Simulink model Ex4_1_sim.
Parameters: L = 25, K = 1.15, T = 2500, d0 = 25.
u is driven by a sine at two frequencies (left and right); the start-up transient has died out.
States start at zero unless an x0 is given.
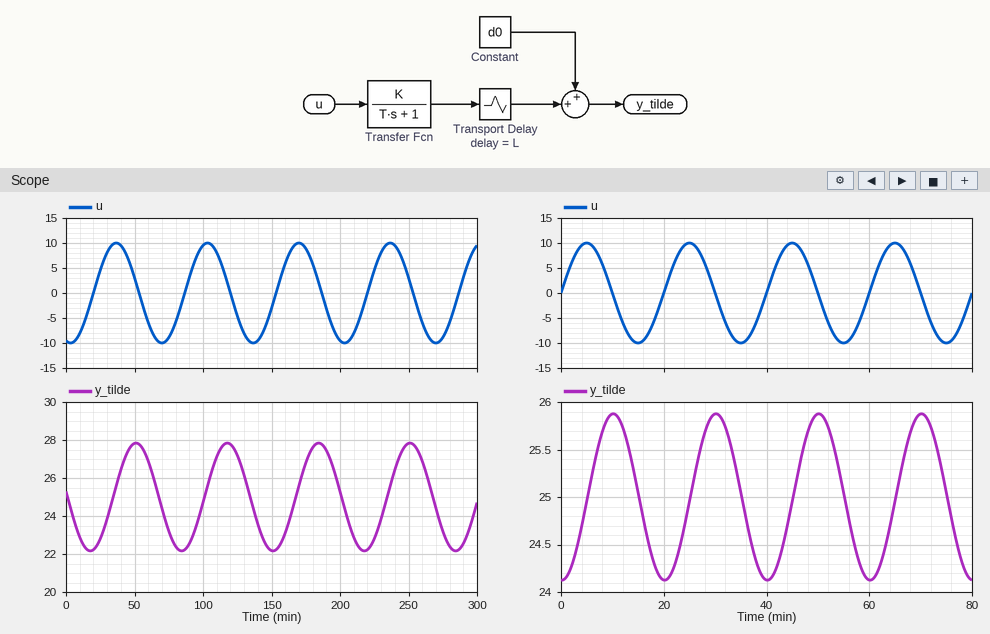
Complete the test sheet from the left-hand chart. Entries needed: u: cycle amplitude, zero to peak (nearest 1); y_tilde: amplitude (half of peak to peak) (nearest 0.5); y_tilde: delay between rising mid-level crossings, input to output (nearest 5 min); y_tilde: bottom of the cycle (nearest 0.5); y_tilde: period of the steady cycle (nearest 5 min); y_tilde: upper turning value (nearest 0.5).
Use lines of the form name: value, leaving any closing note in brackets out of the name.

u: cycle amplitude, zero to peak: 10
y_tilde: amplitude (half of peak to peak): 3.0
y_tilde: delay between rising mid-level crossings, input to output: 15 min
y_tilde: bottom of the cycle: 22.0
y_tilde: period of the steady cycle: 65 min
y_tilde: upper turning value: 28.0
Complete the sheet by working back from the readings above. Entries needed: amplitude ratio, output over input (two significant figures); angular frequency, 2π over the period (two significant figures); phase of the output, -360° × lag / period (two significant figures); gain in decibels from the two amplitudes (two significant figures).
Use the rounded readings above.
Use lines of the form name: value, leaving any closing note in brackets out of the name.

amplitude ratio, output over input: 0.30
angular frequency, 2π over the period: 0.097 rad/min
phase of the output, -360° × lag / period: -83°
gain in decibels from the two amplitudes: -10 dB
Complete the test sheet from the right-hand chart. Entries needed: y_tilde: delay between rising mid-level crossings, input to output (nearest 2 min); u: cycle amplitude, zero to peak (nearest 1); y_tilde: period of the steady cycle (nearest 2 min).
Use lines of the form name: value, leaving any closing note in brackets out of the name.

y_tilde: delay between rising mid-level crossings, input to output: 6 min
u: cycle amplitude, zero to peak: 10
y_tilde: period of the steady cycle: 20 min
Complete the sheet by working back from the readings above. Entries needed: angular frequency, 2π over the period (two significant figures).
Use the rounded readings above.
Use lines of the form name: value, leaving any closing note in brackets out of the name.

angular frequency, 2π over the period: 0.31 rad/min
